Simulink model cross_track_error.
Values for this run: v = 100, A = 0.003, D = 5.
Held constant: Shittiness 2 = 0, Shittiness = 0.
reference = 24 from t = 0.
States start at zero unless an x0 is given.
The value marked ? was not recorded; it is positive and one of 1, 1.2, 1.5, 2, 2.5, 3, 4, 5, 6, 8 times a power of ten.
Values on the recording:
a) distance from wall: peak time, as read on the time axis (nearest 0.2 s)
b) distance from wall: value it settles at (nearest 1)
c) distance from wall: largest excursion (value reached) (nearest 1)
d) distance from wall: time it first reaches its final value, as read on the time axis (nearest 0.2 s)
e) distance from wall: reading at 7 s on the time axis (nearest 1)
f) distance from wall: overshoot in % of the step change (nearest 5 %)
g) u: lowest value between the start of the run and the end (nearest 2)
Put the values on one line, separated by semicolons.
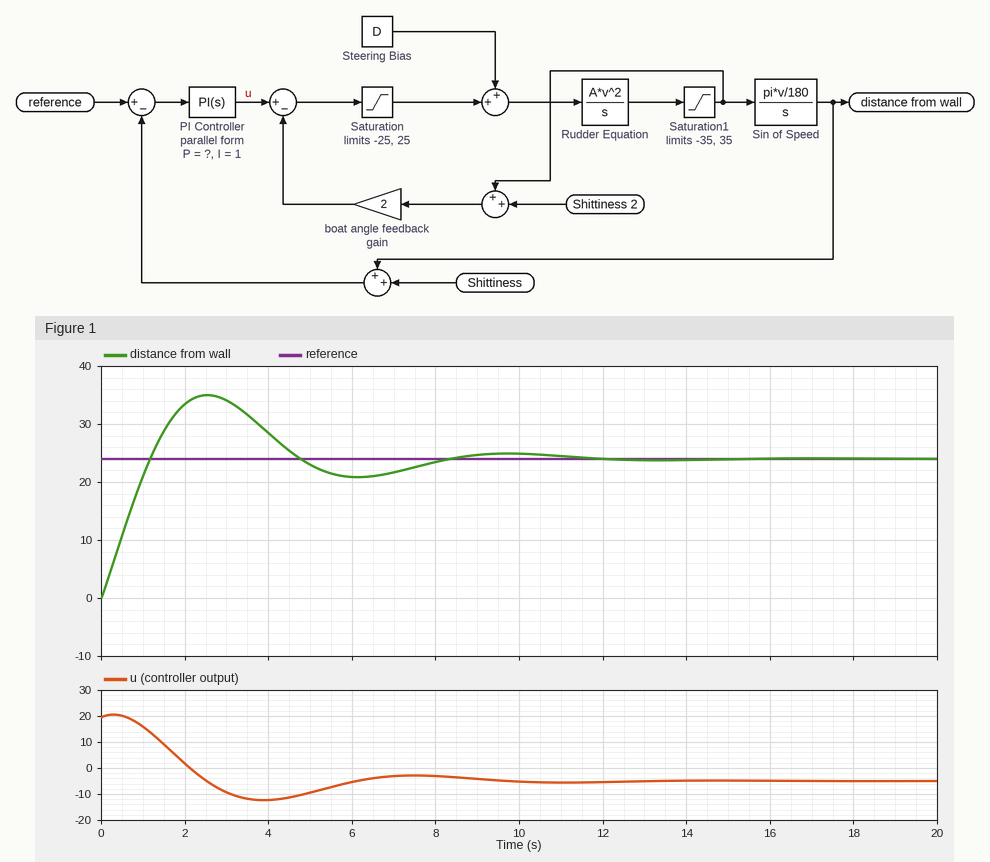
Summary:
2.6 s; 24; 35; 1.2 s; 22; 45 %; -12
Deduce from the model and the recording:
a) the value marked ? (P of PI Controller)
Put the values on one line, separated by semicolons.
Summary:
0.8
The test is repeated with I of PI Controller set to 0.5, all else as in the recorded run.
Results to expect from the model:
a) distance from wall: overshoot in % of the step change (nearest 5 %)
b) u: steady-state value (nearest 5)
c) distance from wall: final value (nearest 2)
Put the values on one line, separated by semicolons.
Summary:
40 %; -5; 24
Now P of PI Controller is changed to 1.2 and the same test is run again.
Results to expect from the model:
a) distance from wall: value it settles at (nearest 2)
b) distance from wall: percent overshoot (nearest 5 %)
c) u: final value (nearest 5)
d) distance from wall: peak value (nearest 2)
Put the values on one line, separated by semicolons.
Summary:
24; 35 %; -5; 32
